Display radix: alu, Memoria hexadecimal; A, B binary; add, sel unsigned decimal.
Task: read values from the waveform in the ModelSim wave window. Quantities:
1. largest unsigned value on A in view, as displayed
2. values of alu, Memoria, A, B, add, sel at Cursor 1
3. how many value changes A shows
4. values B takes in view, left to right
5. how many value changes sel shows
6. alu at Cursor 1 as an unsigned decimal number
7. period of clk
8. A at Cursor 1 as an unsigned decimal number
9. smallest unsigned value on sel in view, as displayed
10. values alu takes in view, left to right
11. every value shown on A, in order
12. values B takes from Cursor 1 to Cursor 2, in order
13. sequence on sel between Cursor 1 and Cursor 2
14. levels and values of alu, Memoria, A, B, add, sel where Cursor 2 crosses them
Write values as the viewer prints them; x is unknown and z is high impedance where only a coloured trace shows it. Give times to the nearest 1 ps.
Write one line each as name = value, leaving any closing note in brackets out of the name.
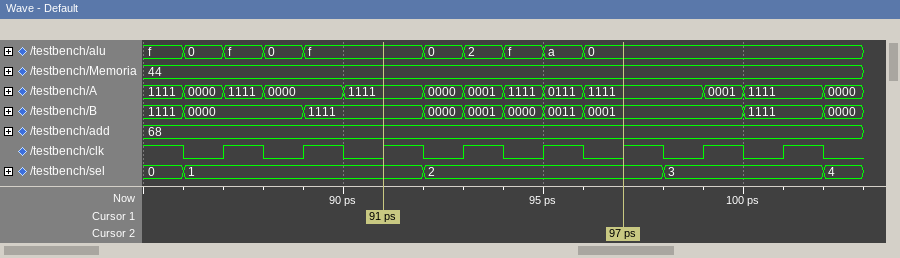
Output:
largest unsigned value on A in view, as displayed = 1111
values of alu, Memoria, A, B, add, sel at Cursor 1 = alu=f, Memoria=44, A=1111, B=1111, add=68, sel=1
how many value changes A shows = 12
values B takes in view, left to right = 1111, 0000, 1111, 0000, 0001, 0000, 0011, 0001, 1111, 0000
how many value changes sel shows = 4
alu at Cursor 1 as an unsigned decimal number = 15
period of clk = 2 ps
A at Cursor 1 as an unsigned decimal number = 15
smallest unsigned value on sel in view, as displayed = 0
values alu takes in view, left to right = f, 0, f, 0, f, 0, 2, f, a, 0
every value shown on A, in order = 1111, 0000, 1111, 0000, 1111, 0000, 0001, 1111, 0111, 1111, 0001, 1111, 0000
values B takes from Cursor 1 to Cursor 2, in order = 1111, 0000, 0001, 0000, 0011, 0001
sequence on sel between Cursor 1 and Cursor 2 = 1, 2
levels and values of alu, Memoria, A, B, add, sel where Cursor 2 crosses them = alu=0, Memoria=44, A=1111, B=0001, add=68, sel=2
